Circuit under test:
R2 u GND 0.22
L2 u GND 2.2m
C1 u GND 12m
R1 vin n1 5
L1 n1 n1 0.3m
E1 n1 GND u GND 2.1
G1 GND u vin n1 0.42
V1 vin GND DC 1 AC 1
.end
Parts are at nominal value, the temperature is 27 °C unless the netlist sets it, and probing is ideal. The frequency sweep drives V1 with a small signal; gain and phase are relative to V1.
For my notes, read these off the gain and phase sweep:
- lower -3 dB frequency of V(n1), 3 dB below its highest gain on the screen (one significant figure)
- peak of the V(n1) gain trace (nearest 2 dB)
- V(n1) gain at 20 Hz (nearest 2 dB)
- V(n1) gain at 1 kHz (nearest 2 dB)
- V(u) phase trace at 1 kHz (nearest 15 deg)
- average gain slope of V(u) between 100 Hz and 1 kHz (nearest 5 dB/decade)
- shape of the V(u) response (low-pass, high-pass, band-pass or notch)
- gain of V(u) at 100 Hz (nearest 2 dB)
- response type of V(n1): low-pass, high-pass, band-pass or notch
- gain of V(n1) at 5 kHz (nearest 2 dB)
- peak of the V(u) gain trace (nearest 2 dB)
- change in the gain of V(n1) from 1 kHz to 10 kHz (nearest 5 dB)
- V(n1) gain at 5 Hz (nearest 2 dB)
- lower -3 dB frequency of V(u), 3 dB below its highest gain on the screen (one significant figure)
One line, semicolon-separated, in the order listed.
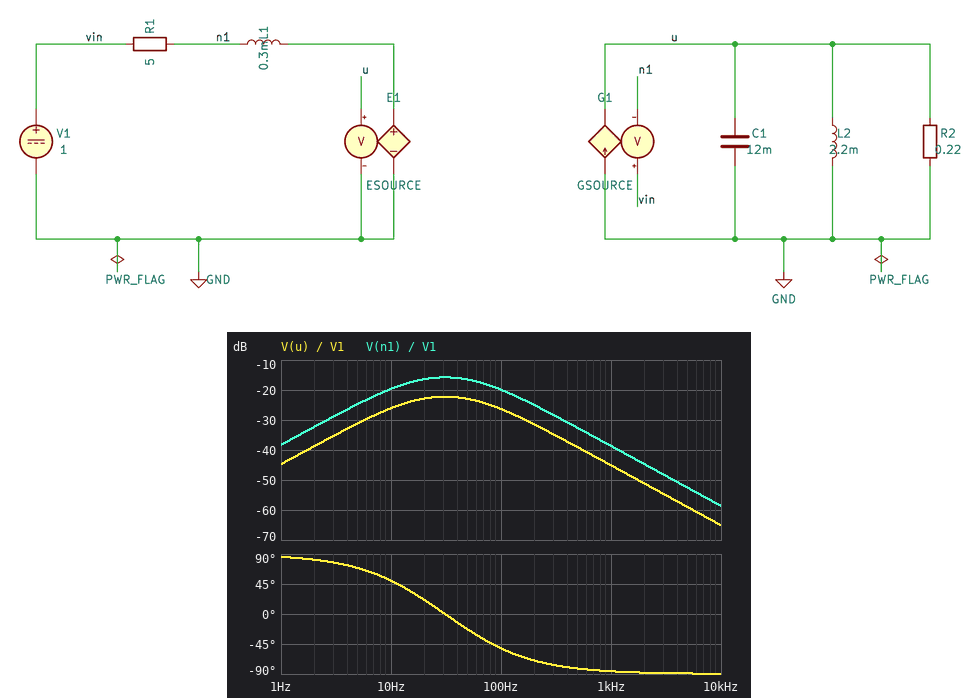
10 Hz; -16 dB; -16 dB; -38 dB; -90 deg; -20 dB/decade; band-pass; -26 dB; band-pass; -52 dB; -22 dB; -20 dB; -24 dB; 10 Hz
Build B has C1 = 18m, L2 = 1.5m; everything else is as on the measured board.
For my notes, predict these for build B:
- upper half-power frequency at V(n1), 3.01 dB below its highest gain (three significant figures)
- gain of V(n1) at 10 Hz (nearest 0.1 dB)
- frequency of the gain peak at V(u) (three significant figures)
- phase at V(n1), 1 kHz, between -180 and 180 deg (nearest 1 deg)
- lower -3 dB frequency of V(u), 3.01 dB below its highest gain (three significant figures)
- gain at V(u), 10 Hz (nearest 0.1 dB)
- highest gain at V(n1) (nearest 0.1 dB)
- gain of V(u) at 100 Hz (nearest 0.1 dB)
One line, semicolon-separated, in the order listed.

62.9 Hz; -21.9 dB; 30.6 Hz; -87 deg; 14.9 Hz; -28.3 dB; -15.8 dB; -28.8 dB
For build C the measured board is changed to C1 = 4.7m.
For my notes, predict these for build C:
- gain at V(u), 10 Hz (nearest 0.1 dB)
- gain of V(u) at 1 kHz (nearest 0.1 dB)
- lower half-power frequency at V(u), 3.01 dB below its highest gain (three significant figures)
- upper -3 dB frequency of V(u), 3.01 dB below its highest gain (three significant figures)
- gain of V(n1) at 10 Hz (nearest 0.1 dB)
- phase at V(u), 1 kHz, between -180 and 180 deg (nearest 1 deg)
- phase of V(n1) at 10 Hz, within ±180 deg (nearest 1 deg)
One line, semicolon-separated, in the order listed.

-26.4 dB; -37.1 dB; 12.5 Hz; 196 Hz; -20.0 dB; -80 deg; 52 deg
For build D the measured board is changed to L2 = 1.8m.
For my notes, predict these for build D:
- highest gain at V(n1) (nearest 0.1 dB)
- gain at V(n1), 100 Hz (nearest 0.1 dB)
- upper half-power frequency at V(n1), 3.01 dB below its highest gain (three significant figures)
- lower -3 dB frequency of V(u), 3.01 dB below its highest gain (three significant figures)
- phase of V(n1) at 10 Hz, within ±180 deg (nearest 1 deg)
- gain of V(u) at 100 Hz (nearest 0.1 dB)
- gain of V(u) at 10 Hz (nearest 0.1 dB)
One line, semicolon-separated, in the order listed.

-15.8 dB; -19.8 dB; 85.7 Hz; 13.7 Hz; 56 deg; -26.2 dB; -27.3 dB
